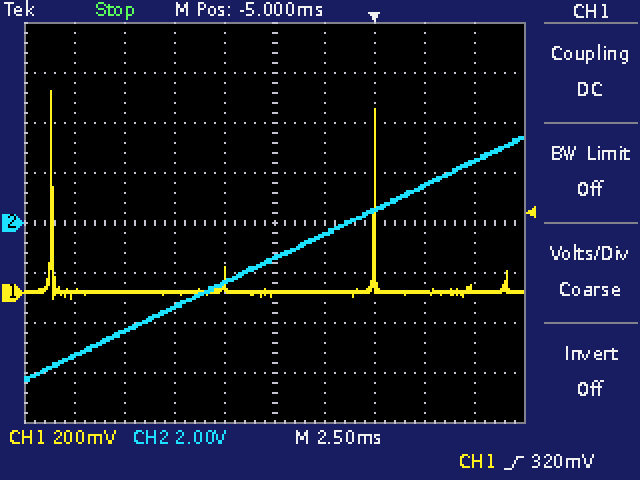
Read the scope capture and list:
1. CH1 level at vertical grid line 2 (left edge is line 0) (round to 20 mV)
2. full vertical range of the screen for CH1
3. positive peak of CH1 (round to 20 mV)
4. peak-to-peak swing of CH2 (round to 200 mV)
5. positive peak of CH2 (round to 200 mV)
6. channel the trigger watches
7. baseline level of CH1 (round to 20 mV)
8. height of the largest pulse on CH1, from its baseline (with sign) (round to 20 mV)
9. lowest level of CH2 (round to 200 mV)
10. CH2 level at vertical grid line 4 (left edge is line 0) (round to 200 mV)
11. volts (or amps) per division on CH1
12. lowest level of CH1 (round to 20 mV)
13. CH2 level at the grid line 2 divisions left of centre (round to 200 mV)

0 mV
1.6 V
800 mV
9.8 V
3.4 V
CH1
0 mV
+800 mV
-6.4 V
-2.4 V
200 mV
-20 mV
-3.4 V
